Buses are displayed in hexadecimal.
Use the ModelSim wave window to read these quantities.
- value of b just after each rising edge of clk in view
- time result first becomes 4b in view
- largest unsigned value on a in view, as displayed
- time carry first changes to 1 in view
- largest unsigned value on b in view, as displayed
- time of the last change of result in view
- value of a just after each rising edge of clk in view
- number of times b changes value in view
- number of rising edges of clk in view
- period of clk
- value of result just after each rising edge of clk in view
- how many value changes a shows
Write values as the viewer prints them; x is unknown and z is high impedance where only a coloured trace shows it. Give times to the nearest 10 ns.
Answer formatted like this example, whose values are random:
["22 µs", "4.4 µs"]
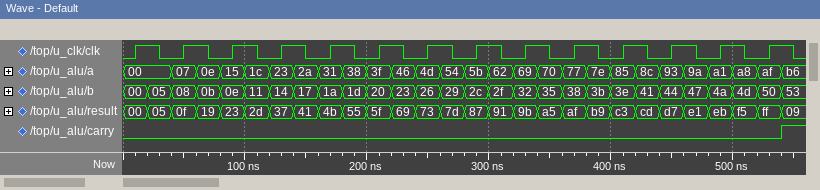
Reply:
["00, 08, 0e, 14, 1a, 20, 26, 2c, 32, 38, 3e, 44, 4a, 50", "160 ns", "b6", "540 ns", "53", "540 ns", "00, 07, 15, 23, 31, 3f, 4d, 5b, 69, 77, 85, 93, a1, af", "27", "14", "40 ns", "00, 0f, 23, 37, 4b, 5f, 73, 87, 9b, af, c3, d7, eb, ff", "26"]
